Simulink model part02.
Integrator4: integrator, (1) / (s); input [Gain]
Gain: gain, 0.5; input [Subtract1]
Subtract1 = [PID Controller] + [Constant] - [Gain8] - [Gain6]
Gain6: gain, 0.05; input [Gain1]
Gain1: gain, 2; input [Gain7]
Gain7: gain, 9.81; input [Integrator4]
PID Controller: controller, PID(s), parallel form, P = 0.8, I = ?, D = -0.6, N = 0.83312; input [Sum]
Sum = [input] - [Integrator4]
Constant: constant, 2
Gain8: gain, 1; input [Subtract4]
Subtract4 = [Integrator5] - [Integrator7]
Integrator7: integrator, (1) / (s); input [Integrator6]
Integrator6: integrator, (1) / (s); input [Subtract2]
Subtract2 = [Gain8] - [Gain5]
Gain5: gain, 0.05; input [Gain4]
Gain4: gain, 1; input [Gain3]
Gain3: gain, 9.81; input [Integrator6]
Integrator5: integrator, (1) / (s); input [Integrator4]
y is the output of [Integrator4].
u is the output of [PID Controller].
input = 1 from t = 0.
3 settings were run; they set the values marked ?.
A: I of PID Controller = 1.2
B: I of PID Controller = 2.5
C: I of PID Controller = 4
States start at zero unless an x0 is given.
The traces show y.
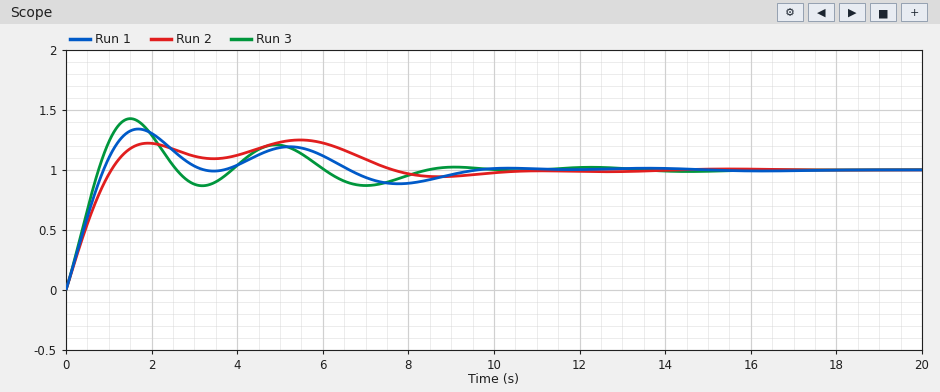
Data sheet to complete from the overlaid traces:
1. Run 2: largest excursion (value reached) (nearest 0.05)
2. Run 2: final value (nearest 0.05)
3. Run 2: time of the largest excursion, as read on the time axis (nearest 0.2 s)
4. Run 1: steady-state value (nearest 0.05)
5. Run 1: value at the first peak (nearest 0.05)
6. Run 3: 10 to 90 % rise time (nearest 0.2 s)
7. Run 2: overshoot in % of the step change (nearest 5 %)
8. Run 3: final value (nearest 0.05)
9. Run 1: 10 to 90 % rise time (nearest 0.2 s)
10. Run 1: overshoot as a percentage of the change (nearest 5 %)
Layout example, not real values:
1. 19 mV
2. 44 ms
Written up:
1. 1.25
2. 1.00
3. 5.4 s
4. 1.00
5. 1.35
6. 0.6 s
7. 25 %
8. 1.00
9. 0.6 s
10. 35 %
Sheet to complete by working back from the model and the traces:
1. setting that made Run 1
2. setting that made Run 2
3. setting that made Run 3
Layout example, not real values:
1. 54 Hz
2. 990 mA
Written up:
1. B
2. A
3. C
